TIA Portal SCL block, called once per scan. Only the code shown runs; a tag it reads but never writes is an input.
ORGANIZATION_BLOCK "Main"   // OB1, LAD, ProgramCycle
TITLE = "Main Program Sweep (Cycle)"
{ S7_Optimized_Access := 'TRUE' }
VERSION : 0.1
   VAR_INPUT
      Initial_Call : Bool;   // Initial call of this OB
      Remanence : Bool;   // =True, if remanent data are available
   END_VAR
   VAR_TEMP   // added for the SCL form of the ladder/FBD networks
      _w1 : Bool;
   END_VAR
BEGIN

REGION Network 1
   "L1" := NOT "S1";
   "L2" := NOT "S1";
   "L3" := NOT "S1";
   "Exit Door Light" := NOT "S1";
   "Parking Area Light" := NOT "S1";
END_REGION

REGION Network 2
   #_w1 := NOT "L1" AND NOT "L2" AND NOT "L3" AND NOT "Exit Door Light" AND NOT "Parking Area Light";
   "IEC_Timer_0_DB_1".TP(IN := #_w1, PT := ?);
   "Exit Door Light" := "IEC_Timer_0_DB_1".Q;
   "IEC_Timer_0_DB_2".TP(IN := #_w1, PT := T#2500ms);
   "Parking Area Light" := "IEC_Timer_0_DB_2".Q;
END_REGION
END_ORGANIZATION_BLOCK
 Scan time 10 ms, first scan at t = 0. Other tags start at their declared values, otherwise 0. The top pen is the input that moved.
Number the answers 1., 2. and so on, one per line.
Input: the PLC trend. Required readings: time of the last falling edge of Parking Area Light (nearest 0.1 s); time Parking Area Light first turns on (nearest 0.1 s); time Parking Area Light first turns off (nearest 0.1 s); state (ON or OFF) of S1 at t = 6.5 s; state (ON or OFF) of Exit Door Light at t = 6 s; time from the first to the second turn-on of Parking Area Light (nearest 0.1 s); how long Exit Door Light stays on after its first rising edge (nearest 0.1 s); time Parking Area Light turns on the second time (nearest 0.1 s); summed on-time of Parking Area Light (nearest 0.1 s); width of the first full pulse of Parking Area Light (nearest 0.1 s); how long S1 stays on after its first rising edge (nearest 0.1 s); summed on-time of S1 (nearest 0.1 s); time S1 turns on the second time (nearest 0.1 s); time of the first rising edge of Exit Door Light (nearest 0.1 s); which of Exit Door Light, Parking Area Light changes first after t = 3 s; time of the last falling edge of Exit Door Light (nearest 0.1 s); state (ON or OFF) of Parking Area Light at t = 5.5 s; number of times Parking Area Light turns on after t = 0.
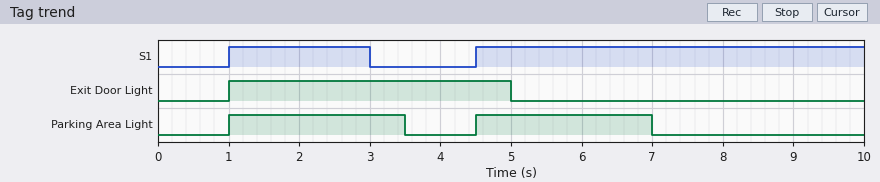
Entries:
1. 7.0 s
2. 1.0 s
3. 3.5 s
4. ON
5. OFF
6. 3.5 s
7. 4.0 s
8. 4.5 s
9. 5.0 s
10. 2.5 s
11. 2.0 s
12. 7.5 s
13. 4.5 s
14. 1.0 s
15. Parking Area Light
16. 5.0 s
17. ON
18. 2
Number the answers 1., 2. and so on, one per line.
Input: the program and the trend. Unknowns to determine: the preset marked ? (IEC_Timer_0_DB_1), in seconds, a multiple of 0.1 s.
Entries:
1. 4.0 s
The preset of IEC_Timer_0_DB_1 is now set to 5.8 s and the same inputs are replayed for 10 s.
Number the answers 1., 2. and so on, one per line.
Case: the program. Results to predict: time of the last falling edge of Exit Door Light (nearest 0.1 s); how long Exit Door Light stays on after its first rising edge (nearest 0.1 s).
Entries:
1. 6.8 s
2. 5.8 s
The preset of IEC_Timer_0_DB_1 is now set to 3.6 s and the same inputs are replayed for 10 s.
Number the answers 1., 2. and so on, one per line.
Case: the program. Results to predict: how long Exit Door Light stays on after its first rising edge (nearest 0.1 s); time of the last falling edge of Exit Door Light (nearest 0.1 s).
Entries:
1. 3.6 s
2. 4.6 s
